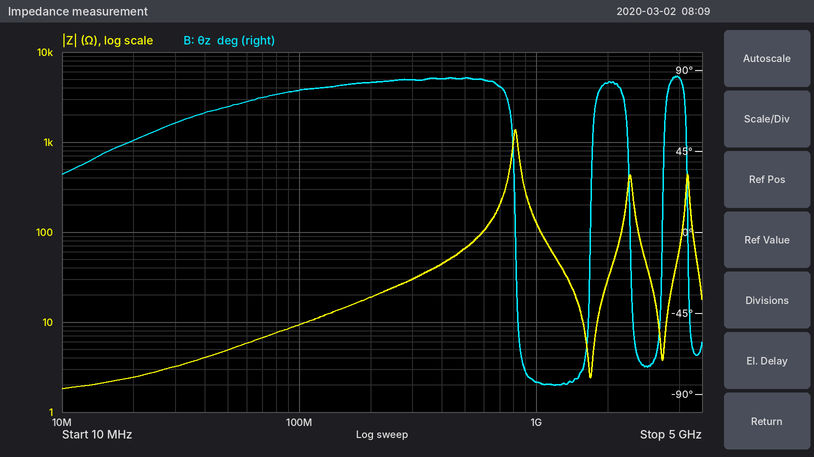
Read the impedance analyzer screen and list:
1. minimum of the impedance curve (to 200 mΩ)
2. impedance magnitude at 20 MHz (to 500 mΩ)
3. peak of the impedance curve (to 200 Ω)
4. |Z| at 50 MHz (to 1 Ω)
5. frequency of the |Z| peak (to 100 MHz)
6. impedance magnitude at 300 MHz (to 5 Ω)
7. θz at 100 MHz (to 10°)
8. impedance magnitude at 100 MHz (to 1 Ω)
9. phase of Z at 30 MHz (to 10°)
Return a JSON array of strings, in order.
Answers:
["1.8 Ω", "2.5 Ω", "1.4 kΩ", "5 Ω", "800 MHz", "30 Ω", "80°", "9 Ω", "60°"]
